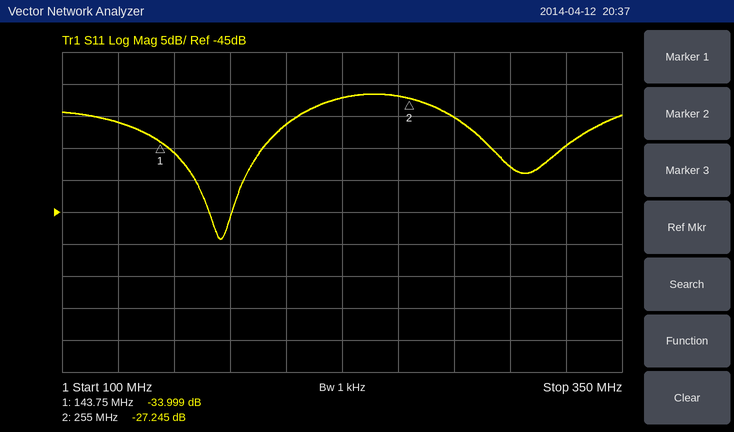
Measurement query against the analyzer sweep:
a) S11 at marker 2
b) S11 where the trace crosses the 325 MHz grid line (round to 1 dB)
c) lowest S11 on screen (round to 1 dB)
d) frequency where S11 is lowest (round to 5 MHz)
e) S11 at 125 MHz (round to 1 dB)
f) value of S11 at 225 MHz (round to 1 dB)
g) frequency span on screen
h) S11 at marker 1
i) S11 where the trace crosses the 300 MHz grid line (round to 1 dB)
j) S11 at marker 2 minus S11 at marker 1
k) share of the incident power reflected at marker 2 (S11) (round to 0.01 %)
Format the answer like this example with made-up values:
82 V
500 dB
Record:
-27.245 dB
-35 dB
-49 dB
170 MHz
-31 dB
-27 dB
250 MHz
-33.999 dB
-38 dB
6.754 dB
0.19 %
